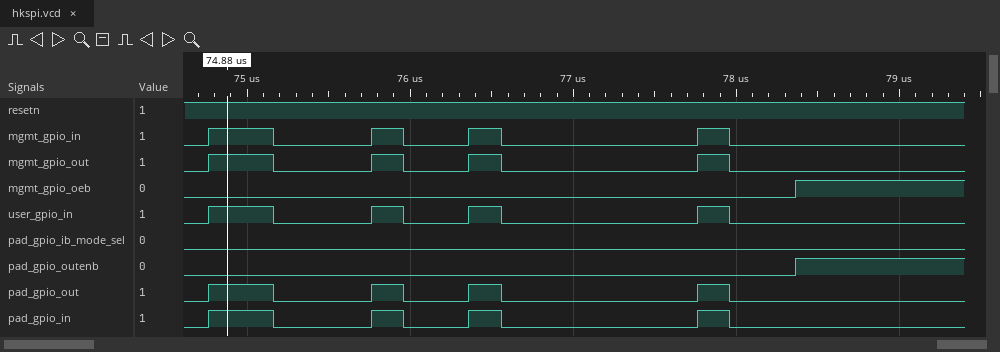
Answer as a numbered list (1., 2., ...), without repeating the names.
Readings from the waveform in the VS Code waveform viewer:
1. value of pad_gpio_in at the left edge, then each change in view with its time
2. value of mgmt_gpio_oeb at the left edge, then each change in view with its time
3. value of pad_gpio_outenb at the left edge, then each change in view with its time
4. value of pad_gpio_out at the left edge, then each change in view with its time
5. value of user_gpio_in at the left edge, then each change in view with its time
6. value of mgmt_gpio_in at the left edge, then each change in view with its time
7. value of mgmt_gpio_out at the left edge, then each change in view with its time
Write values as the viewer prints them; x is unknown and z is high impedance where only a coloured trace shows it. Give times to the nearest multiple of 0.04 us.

1. 0, 1 at 74.76 us, 0 at 75.16 us, 1 at 75.76 us, 0 at 75.96 us, 1 at 76.36 us, 0 at 76.56 us, 1 at 77.76 us, 0 at 77.96 us
2. 0, 1 at 78.36 us
3. 0, 1 at 78.36 us
4. 0, 1 at 74.76 us, 0 at 75.16 us, 1 at 75.76 us, 0 at 75.96 us, 1 at 76.36 us, 0 at 76.56 us, 1 at 77.76 us, 0 at 77.96 us
5. 0, 1 at 74.76 us, 0 at 75.16 us, 1 at 75.76 us, 0 at 75.96 us, 1 at 76.36 us, 0 at 76.56 us, 1 at 77.76 us, 0 at 77.96 us
6. 0, 1 at 74.76 us, 0 at 75.16 us, 1 at 75.76 us, 0 at 75.96 us, 1 at 76.36 us, 0 at 76.56 us, 1 at 77.76 us, 0 at 77.96 us
7. 0, 1 at 74.76 us, 0 at 75.16 us, 1 at 75.76 us, 0 at 75.96 us, 1 at 76.36 us, 0 at 76.56 us, 1 at 77.76 us, 0 at 77.96 us
